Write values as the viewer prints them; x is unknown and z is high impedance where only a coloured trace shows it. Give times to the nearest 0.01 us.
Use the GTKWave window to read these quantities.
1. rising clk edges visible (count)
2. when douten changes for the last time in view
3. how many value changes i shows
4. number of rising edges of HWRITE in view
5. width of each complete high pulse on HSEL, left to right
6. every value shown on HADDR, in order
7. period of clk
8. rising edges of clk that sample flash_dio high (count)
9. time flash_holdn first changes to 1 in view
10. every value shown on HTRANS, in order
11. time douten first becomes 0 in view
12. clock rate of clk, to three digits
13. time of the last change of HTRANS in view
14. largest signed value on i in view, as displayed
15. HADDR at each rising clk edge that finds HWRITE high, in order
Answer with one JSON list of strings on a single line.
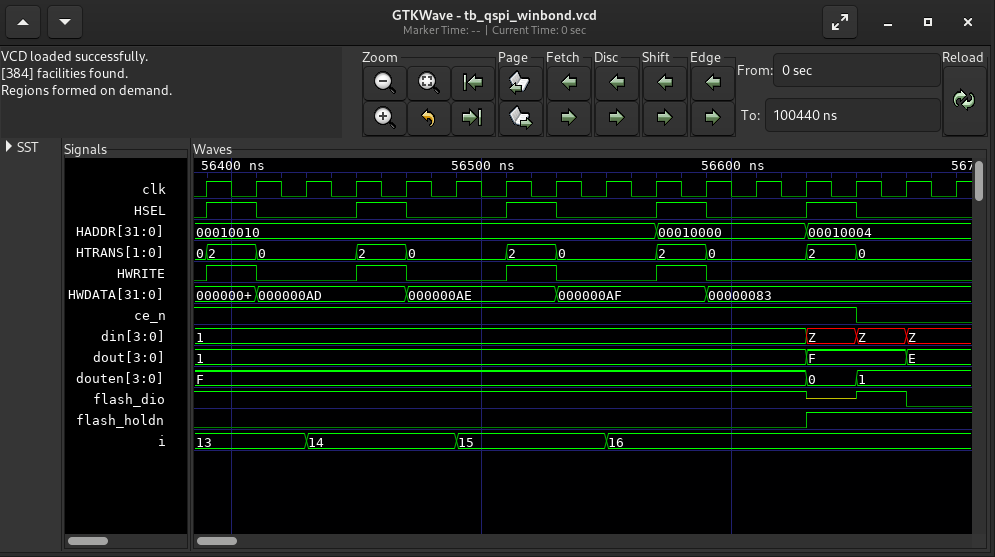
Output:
["16", "56.65 us", "3", "4", "0.02 us, 0.02 us, 0.02 us, 0.02 us, 0.02 us", "00010010, 00010000, 00010004", "0.02 us", "14", "56.63 us", "0, 2, 0, 2, 0, 2, 0, 2, 0, 2, 0", "56.63 us", "50.0 MHz", "56.65 us", "16", "00010010, 00010010, 00010010, 00010000"]
